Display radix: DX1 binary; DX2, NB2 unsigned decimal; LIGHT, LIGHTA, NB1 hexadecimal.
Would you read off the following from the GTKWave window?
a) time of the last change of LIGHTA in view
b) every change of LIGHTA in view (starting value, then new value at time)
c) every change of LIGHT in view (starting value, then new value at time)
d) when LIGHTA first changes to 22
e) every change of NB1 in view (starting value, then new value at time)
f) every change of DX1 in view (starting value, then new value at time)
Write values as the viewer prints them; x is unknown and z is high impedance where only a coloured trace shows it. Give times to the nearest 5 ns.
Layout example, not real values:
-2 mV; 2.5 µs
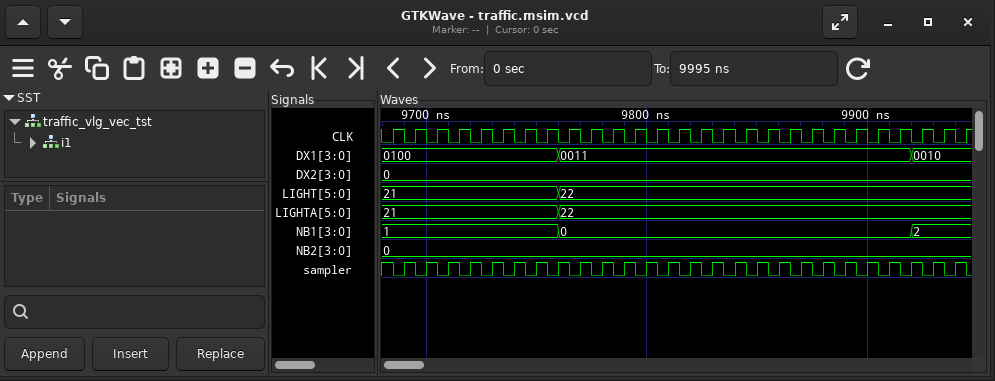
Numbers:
9760 ns; 21, 22 at 9760 ns; 21, 22 at 9760 ns; 9760 ns; 1, 0 at 9760 ns, 2 at 9920 ns; 0100, 0011 at 9760 ns, 0010 at 9920 ns
